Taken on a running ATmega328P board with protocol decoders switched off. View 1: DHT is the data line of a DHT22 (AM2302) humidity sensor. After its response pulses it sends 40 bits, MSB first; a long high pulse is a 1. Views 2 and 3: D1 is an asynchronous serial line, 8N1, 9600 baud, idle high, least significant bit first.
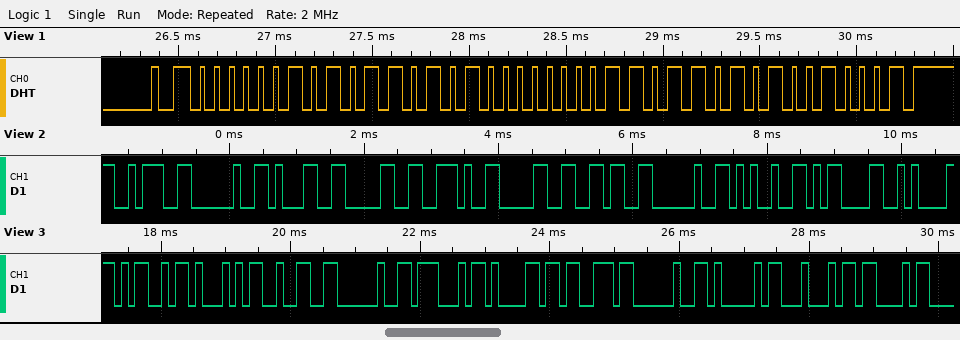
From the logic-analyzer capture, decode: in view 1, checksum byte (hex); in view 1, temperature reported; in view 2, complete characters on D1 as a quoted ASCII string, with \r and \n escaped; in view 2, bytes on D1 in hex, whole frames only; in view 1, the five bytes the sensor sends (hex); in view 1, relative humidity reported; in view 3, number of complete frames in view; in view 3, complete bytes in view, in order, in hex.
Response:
0x91
21.8 °C
": 10.06 %\r\n"
3A 20 31 30 2E 30 36 20 25 0D 0A
02 B5 00 DA 91
69.3 %
11
4D 51 32 20 47 61 73 20 41 44 43
